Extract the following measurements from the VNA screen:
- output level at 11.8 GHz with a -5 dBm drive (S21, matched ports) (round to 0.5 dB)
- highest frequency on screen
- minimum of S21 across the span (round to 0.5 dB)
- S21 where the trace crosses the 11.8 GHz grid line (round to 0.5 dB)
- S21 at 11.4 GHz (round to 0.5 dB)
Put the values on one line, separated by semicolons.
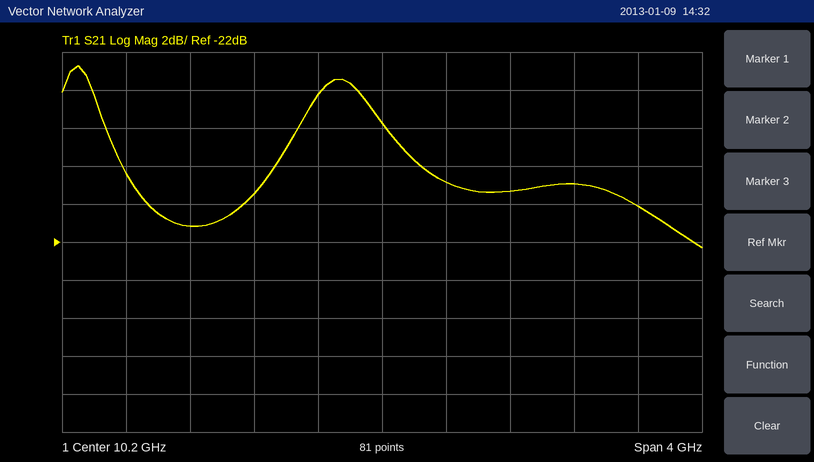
-25.0 dBm; 12.2 GHz; -22.5 dB; -20.0 dB; -19.0 dB
